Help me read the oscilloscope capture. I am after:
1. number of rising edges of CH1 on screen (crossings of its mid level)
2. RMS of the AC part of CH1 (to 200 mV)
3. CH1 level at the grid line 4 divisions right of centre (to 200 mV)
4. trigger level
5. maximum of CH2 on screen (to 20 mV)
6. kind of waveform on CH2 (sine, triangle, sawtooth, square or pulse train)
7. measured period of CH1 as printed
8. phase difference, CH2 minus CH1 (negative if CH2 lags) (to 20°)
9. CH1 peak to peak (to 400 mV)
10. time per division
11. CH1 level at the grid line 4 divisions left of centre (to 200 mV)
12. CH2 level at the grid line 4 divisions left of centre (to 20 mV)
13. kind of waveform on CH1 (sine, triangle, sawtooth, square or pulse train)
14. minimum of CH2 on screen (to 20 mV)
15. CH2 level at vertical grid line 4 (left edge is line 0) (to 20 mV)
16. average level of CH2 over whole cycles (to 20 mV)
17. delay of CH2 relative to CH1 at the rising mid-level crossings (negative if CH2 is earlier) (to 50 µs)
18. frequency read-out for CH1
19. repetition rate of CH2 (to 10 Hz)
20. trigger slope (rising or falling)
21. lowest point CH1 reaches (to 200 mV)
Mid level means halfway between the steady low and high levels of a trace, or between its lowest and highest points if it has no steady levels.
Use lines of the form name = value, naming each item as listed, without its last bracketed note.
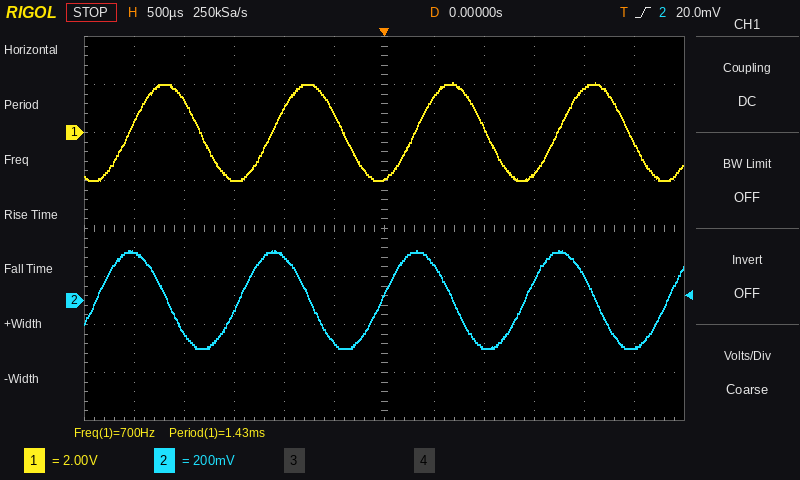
number of rising edges of CH1 on screen = 4
RMS of the AC part of CH1 = 1.4 V
CH1 level at the grid line 4 divisions right of centre = 1.8 V
trigger level = 20.0 mV
maximum of CH2 on screen = 200 mV
kind of waveform on CH2 = sine
measured period of CH1 as printed = 1.43 ms
phase difference, CH2 minus CH1 (negative if CH2 lags) = +80°
CH1 peak to peak = 4.0 V
time per division = 500 µs
CH1 level at the grid line 4 divisions left of centre = 1.4 V
CH2 level at the grid line 4 divisions left of centre = -140 mV
kind of waveform on CH1 = sine
minimum of CH2 on screen = -200 mV
CH2 level at vertical grid line 4 (left edge is line 0) = 180 mV
average level of CH2 over whole cycles = 0 mV
delay of CH2 relative to CH1 at the rising mid-level crossings (negative if CH2 is earlier) = -350 µs
frequency read-out for CH1 = 700 Hz
repetition rate of CH2 = 700 Hz
trigger slope = rising
lowest point CH1 reaches = -2.0 V
